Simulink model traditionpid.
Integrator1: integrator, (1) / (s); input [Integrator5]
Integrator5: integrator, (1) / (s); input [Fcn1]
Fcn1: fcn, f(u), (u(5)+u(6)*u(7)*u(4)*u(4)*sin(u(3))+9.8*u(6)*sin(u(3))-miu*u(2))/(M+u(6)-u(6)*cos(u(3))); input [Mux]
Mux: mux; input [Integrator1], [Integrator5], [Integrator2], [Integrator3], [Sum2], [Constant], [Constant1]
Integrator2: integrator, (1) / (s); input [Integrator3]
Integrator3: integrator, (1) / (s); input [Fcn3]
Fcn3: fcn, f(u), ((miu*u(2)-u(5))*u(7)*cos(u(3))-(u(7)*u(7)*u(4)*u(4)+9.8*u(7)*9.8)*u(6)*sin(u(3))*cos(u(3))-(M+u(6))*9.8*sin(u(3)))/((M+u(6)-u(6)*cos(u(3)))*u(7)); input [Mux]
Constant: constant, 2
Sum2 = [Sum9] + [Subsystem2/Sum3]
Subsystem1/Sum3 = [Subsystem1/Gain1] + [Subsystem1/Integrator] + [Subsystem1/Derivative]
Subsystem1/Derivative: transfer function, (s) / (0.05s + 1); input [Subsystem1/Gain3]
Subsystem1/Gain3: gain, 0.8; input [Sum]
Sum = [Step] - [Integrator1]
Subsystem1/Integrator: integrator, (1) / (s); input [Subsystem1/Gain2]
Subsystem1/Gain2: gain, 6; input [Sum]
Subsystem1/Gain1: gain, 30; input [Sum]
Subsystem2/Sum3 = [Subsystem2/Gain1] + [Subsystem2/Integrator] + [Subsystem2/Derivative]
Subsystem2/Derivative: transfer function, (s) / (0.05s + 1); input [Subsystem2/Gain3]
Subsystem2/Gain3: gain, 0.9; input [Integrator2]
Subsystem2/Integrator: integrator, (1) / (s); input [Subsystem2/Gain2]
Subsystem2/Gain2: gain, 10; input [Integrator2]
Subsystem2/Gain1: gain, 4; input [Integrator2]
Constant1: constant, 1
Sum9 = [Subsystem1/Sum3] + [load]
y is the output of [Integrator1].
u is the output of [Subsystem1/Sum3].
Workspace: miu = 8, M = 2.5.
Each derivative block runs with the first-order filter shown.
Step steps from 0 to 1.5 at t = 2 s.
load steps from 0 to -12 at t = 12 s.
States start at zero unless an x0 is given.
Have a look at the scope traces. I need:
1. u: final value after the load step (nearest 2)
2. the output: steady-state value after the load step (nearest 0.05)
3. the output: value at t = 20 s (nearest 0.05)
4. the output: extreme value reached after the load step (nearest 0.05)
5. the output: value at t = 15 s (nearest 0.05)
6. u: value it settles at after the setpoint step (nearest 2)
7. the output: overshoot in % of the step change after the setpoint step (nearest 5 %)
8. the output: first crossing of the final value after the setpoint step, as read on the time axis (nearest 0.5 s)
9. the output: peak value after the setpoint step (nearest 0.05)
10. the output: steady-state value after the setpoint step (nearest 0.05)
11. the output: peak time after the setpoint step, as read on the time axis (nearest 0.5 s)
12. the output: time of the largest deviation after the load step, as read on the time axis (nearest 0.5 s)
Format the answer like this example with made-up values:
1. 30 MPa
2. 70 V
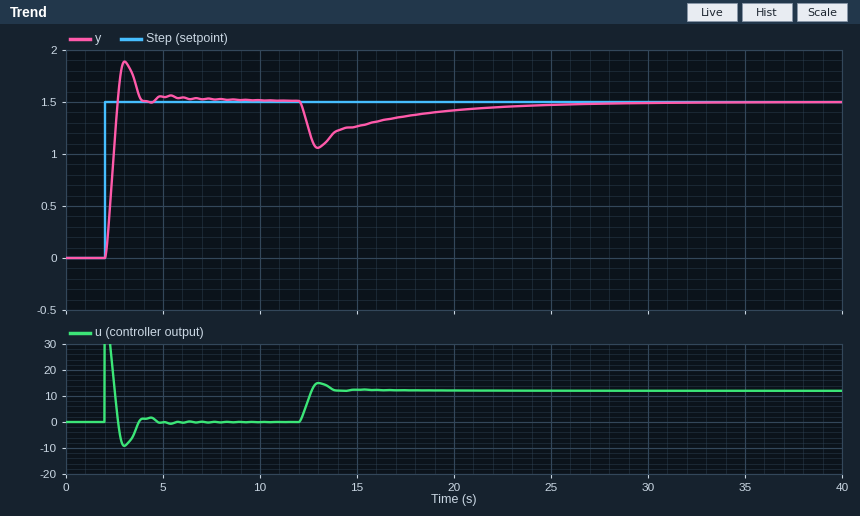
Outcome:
1. 12
2. 1.50
3. 1.40
4. 1.05
5. 1.25
6. 0
7. 25 %
8. 2.5 s
9. 1.90
10. 1.50
11. 3.0 s
12. 13.0 s
